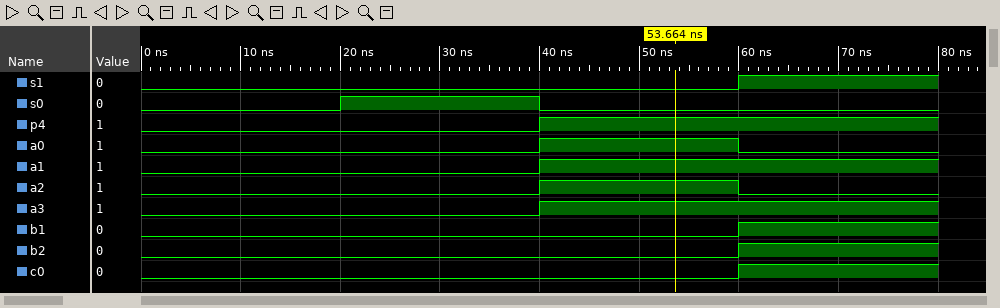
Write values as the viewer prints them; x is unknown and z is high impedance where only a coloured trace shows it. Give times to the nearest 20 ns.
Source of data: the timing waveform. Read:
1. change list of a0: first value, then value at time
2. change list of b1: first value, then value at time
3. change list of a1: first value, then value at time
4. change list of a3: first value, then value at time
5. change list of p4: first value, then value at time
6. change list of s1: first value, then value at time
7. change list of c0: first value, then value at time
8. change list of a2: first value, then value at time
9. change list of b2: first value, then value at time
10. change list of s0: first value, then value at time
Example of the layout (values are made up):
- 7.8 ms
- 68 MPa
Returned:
- 0, 1 at 40 ns, 0 at 60 ns
- 0, 1 at 60 ns
- 0, 1 at 40 ns
- 0, 1 at 40 ns
- 0, 1 at 40 ns
- 0, 1 at 60 ns
- 0, 1 at 60 ns
- 0, 1 at 40 ns, 0 at 60 ns
- 0, 1 at 60 ns
- 0, 1 at 20 ns, 0 at 40 ns
